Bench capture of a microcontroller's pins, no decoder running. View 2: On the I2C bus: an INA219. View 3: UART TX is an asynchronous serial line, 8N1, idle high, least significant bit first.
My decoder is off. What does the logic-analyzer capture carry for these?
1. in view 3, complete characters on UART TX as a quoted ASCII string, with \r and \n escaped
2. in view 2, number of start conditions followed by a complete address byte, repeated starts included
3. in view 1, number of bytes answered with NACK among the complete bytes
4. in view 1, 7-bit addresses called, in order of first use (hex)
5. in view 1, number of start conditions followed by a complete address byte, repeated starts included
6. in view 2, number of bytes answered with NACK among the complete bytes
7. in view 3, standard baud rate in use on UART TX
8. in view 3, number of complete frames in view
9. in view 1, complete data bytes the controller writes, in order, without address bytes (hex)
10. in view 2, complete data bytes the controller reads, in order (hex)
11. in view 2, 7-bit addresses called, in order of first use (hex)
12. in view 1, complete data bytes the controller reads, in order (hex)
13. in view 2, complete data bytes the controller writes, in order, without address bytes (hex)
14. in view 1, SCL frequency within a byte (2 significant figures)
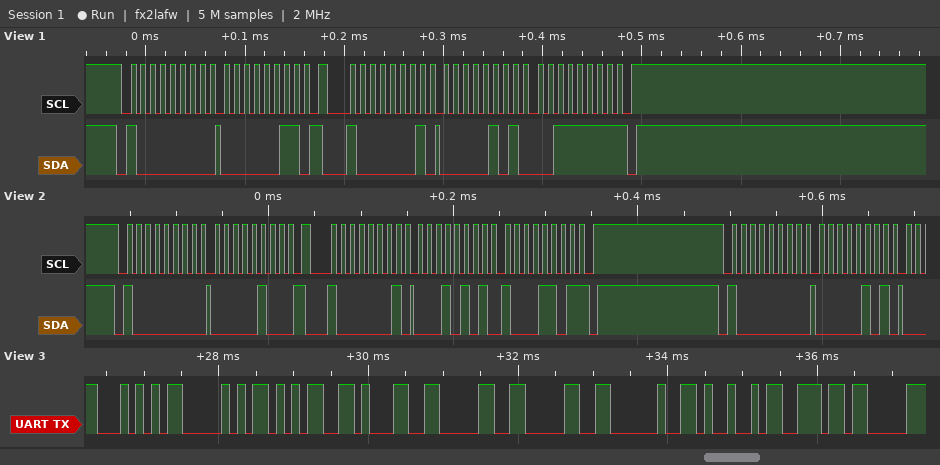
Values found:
"TP5100 In"
3
1
0x40
2
1
9600 baud
9
03
15 8D
0x40
05 3F
04 05
100 kHz
